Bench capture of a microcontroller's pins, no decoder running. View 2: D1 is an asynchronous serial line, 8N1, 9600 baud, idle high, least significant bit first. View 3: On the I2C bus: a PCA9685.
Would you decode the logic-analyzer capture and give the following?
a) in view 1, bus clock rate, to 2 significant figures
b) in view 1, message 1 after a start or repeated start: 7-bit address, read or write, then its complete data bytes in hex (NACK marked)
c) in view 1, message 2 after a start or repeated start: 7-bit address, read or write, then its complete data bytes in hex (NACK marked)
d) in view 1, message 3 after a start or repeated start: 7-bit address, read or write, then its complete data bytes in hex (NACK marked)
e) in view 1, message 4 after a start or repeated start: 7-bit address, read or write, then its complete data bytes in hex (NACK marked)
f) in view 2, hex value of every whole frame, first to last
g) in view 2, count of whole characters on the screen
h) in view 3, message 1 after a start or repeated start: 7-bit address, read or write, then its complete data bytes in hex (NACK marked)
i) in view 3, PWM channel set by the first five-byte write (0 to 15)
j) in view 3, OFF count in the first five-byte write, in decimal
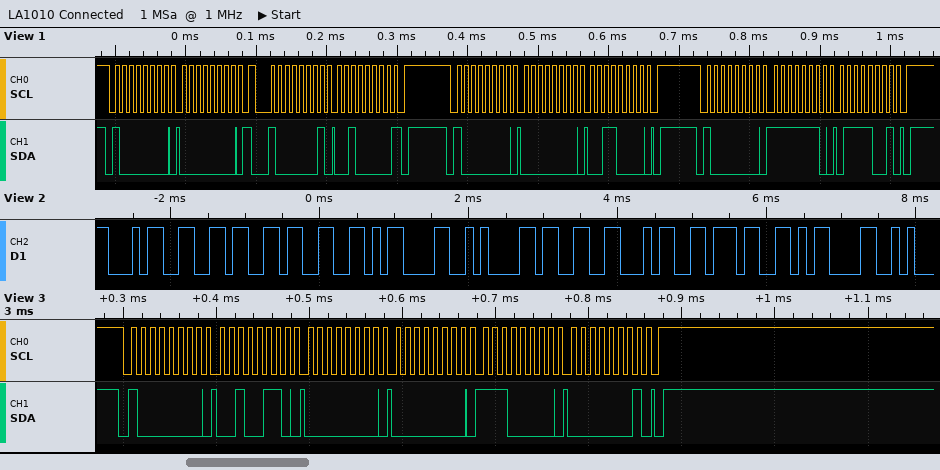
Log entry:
100 kHz
0x40 write: 00
0x40 read: 20 NACK
0x40 write: 00 30
0x40 write: FE 79
34 36 33 0D 0A 33 34 37 0D
9
0x40 write: 26 00 00 E0 01
8
480
